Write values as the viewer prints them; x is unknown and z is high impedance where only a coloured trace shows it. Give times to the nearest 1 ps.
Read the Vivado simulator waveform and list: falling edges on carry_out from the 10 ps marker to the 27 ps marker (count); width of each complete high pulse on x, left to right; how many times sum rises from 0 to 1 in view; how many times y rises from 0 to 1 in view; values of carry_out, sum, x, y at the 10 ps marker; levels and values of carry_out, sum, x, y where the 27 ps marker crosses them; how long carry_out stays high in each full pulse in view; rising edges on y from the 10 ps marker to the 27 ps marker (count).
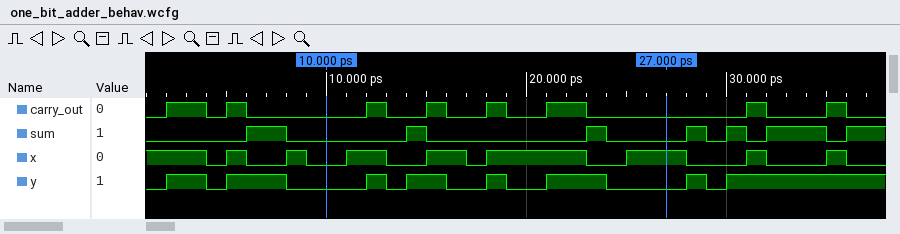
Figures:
4
1 ps, 1 ps, 2 ps, 2 ps, 5 ps, 3 ps, 1 ps, 1 ps
7
8
carry_out=0, sum=0, x=0, y=0
carry_out=0, sum=0, x=1, y=0
2 ps, 1 ps, 1 ps, 1 ps, 1 ps, 2 ps, 1 ps, 1 ps
4
